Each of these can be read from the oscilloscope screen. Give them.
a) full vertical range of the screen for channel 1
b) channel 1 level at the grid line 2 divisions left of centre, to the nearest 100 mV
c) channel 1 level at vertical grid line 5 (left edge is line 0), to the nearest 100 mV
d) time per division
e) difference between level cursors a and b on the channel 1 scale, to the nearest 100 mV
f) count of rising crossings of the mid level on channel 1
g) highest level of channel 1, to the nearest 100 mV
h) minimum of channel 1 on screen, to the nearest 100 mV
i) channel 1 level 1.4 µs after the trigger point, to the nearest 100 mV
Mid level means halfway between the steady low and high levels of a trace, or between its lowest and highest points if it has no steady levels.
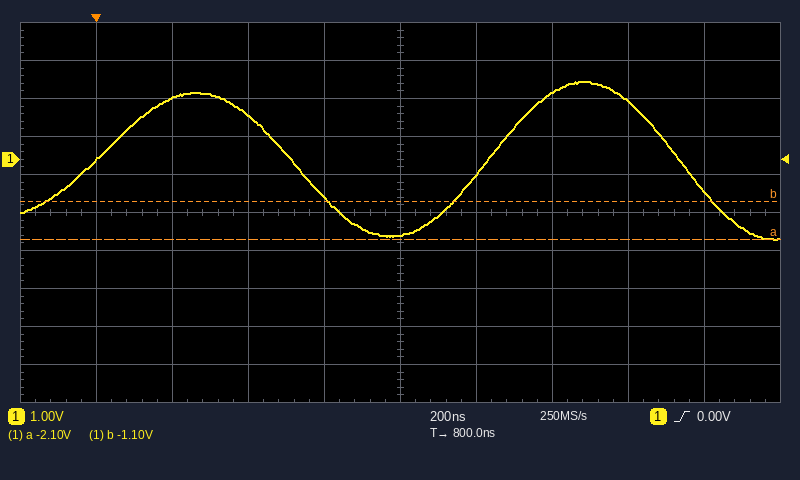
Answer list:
10 V
1.2 V
-2.0 V
200 ns
1.0 V
2
2.0 V
-2.1 V
1.5 V
